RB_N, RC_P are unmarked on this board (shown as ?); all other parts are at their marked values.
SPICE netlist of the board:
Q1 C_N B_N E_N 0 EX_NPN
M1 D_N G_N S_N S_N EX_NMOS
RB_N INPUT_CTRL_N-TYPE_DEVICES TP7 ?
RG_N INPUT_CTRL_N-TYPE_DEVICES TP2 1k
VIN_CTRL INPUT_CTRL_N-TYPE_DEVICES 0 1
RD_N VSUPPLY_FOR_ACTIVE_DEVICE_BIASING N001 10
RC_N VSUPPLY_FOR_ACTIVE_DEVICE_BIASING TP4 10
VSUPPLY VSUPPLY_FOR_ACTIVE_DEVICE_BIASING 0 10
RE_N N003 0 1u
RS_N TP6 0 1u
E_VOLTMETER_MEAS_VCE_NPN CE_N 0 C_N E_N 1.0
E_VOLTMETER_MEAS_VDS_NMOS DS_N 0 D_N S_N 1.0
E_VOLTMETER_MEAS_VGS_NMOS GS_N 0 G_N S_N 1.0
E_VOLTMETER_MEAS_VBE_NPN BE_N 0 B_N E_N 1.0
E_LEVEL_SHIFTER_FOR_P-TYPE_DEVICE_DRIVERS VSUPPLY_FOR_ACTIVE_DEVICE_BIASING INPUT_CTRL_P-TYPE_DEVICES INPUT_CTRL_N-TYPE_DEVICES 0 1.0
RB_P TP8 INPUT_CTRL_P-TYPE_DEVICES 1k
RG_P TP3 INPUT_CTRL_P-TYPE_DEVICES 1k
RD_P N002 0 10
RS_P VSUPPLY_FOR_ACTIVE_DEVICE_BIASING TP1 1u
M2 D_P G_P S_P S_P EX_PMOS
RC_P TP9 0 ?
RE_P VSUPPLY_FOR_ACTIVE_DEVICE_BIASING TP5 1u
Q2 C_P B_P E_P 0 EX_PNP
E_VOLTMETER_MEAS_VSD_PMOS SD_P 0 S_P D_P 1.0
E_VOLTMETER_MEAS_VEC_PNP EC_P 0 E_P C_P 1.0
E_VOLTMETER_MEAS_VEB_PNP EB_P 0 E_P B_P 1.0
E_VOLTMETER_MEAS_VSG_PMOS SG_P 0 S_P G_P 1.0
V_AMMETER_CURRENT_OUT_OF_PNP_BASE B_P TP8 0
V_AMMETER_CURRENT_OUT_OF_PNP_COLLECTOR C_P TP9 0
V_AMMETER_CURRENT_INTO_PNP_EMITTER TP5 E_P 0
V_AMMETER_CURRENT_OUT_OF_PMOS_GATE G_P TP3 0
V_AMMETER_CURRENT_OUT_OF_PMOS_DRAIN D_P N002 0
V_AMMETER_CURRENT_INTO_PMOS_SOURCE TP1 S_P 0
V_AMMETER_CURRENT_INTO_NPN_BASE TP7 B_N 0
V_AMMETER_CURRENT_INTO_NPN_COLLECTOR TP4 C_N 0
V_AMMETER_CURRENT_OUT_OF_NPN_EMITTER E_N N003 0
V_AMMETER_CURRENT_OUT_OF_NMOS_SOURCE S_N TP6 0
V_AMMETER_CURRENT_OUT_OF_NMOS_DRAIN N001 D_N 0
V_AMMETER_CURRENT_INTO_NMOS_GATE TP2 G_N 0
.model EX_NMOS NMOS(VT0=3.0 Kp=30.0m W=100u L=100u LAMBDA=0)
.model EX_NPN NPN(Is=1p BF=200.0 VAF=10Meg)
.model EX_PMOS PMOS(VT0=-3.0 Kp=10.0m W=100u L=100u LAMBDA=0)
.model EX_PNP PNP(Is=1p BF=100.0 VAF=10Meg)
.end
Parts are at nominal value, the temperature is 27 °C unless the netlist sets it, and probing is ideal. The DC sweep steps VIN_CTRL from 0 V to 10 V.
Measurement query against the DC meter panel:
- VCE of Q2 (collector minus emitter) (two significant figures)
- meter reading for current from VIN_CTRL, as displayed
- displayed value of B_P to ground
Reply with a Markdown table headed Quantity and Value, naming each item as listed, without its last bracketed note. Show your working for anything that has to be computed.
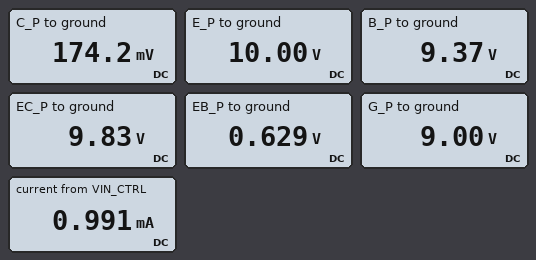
| Quantity | Value |
|---|---|
| VCE of Q2 (collector minus emitter) | 174.2 mV - 10 V = -9.8 V |
| meter reading for current from VIN_CTRL, as displayed | 0.991 mA |
| displayed value of B_P to ground | 9.37 V |
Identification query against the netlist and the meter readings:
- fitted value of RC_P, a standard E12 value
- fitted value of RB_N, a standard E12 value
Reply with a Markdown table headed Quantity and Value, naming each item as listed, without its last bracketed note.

| Quantity | Value |
|---|---|
| fitted value of RC_P, a standard E12 value | 4.7 Ω |
| fitted value of RB_N, a standard E12 value | 330 Ω |
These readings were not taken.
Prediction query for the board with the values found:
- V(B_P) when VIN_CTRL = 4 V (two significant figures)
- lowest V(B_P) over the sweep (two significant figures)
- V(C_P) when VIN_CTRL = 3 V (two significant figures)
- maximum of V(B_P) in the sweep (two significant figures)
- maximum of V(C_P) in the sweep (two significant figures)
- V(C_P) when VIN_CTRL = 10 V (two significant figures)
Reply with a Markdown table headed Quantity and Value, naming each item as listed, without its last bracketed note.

| Quantity | Value |
|---|---|
| V(B_P) when VIN_CTRL = 4 V | 9.3 V |
| lowest V(B_P) over the sweep | 9.3 V |
| V(C_P) when VIN_CTRL = 3 V | 1.1 V |
| maximum of V(B_P) in the sweep | 10 V |
| maximum of V(C_P) in the sweep | 4.4 V |
| V(C_P) when VIN_CTRL = 10 V | 4.4 V |
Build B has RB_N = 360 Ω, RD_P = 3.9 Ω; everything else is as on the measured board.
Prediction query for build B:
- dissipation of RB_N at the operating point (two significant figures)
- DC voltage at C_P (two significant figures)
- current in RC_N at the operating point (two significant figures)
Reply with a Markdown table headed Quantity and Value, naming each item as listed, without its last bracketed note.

| Quantity | Value |
|---|---|
| dissipation of RB_N at the operating point | 300 µW |
| DC voltage at C_P | 170 mV |
| current in RC_N at the operating point | 180 mA |
